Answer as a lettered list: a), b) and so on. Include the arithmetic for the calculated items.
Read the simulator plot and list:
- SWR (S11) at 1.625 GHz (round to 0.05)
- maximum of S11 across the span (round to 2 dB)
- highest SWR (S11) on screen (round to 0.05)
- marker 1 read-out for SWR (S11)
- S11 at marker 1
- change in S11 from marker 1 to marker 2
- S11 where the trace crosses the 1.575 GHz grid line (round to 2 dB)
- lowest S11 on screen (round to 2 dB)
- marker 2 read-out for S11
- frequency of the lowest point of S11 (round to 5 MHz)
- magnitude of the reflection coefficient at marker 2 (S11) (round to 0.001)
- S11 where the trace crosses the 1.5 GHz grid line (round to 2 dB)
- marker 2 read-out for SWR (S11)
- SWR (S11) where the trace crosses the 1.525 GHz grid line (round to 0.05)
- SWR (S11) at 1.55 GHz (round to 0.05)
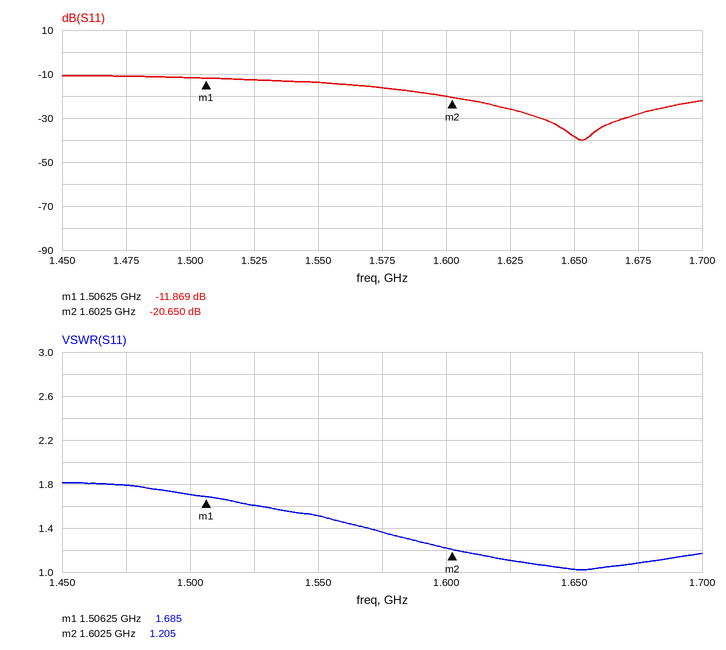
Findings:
a) 1.10
b) -10 dB
c) 1.80
d) 1.685
e) -11.869 dB
f) -20.65 − (-11.869) = -8.781 dB
g) -16 dB
h) -40 dB
i) -20.650 dB
j) 1.655 GHz
k) 10^(-20.65/20) ≈ 0.093
l) -12 dB
m) 1.205
n) 1.60
o) 1.50
